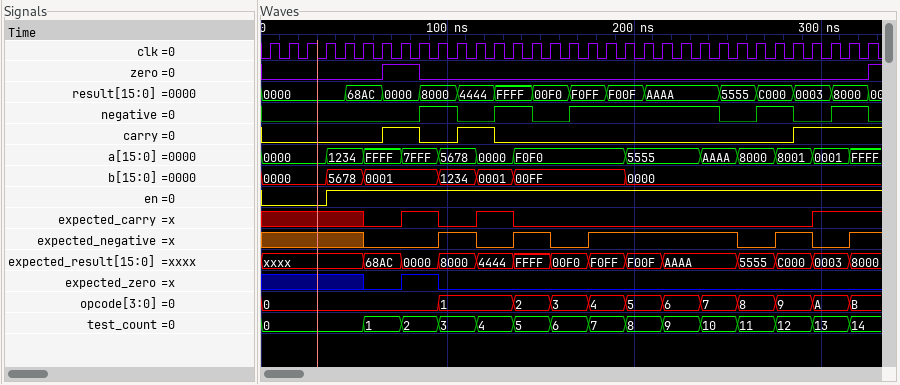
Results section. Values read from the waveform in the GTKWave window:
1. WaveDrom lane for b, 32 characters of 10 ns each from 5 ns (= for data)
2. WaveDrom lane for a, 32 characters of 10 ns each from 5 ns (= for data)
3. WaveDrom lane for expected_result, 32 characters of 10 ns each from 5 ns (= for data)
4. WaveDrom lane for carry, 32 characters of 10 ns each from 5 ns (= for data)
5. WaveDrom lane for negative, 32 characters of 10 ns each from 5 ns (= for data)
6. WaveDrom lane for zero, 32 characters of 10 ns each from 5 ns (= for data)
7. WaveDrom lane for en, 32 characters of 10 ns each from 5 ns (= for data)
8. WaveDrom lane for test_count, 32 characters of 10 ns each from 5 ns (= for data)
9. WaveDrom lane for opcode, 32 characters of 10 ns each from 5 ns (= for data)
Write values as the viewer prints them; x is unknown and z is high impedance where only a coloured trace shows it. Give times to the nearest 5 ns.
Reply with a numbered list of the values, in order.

1. {name: 'b', wave: '=..=.=...=.=.=.....=............', data: '0000 5678 0001 1234 0001 00FF 0000'}
2. {name: 'a', wave: '=..=.=.=.=.=.=.....=...=.=.=.=.=', data: '0000 1234 FFFF 7FFF 5678 0000 F0F0 5555 AAAA 8000 8001 0001 FFFF'}
3. {name: 'expected_result', wave: 'x....=.=.=.=.=.=.=.=.=...=.=.=.=', data: '68AC 0000 8000 4444 FFFF 00F0 F0FF F00F AAAA 5555 C000 0003 8000'}
4. {name: 'carry', wave: '0.....1.0.1.0...............1...'}
5. {name: 'negative', wave: '0.......1.0.1.0.1.......0.1.0.1.'}
6. {name: 'zero', wave: '0.....1.0.......................'}
7. {name: 'en', wave: '0..1............................'}
8. {name: 'test_count', wave: '=....=.=.=.=.=.=.=.=.=.=.=.=.=.=', data: '0 1 2 3 4 5 6 7 8 9 10 11 12 13 14'}
9. {name: 'opcode', wave: '=........=...=.=.=.=.=.=.=.=.=.=', data: '0 1 2 3 4 5 6 7 8 9 A B'}
